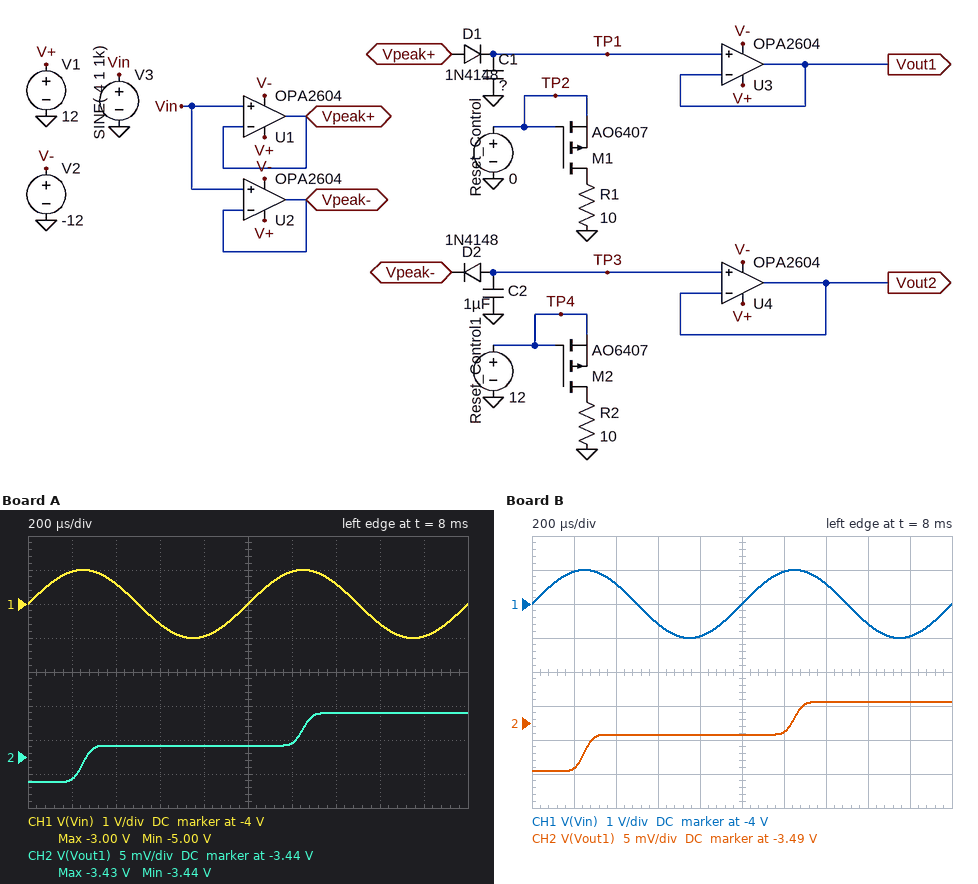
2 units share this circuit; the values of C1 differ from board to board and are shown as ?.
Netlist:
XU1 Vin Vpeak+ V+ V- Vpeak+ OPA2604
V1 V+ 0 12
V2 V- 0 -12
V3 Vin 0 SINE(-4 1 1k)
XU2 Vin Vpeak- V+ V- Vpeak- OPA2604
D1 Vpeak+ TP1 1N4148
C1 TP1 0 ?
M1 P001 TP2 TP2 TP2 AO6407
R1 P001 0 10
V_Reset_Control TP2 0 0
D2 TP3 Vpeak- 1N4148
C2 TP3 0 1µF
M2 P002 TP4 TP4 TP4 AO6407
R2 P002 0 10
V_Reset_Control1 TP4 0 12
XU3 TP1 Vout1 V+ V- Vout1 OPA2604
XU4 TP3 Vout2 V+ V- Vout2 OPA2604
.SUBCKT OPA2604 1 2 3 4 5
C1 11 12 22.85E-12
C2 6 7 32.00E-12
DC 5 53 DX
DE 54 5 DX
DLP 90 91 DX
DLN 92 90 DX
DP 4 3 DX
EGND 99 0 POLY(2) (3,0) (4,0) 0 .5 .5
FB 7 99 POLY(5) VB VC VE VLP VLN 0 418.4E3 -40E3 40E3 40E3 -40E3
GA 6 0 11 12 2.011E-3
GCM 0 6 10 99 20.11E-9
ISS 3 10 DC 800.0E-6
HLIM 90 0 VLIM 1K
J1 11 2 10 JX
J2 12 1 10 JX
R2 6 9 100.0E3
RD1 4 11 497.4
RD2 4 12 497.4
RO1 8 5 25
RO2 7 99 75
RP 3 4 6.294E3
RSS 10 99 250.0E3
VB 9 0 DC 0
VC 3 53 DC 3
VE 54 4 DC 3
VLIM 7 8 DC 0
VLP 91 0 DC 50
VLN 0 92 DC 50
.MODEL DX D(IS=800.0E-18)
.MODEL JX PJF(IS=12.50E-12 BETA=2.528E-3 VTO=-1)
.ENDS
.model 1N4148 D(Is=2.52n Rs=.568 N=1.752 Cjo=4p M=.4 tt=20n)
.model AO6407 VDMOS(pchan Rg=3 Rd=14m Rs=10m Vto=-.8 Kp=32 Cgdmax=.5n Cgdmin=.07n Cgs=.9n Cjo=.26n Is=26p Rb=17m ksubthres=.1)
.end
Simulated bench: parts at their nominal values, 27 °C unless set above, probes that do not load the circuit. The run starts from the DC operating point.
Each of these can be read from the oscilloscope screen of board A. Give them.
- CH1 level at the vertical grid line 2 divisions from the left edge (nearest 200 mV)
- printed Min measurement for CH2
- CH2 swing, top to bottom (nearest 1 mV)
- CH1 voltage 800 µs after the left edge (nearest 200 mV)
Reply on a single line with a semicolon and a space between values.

-3.4 V; -3.44 V; 10 mV; -5.0 V
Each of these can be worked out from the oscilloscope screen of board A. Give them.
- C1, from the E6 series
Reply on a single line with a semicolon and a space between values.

680 nF
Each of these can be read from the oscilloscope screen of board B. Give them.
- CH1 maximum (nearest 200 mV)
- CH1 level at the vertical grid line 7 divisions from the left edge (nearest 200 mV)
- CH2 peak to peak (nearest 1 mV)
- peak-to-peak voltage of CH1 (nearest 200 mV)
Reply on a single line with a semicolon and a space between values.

-3.0 V; -3.4 V; 10 mV; 2.0 V
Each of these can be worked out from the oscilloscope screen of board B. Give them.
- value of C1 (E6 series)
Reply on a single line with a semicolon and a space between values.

2.2 µF
